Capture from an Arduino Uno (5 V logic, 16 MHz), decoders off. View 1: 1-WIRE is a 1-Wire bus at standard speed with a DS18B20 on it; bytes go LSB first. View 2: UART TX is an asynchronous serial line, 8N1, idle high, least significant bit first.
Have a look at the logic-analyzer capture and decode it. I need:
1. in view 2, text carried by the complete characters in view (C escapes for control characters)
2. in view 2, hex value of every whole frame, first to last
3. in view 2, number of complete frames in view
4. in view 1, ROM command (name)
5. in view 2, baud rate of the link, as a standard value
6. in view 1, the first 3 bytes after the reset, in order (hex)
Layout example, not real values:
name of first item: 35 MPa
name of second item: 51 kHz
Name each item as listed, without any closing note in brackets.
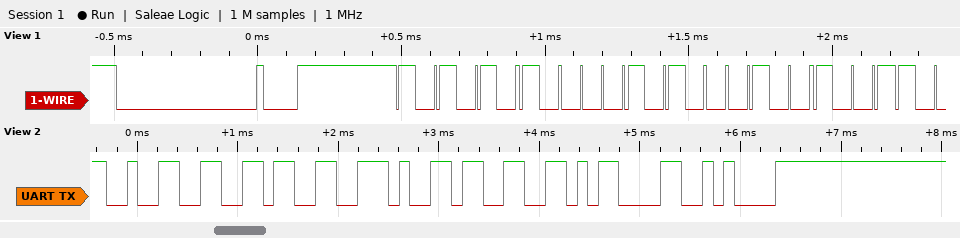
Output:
in view 2, text carried by the complete characters in view: "26.3\r\n"
in view 2, hex value of every whole frame, first to last: 32 36 2E 33 0D 0A
in view 2, number of complete frames in view: 6
in view 1, ROM command: Match ROM
in view 2, baud rate of the link, as a standard value: 9600 baud
in view 1, the first 3 bytes after the reset, in order: 55 28 92
